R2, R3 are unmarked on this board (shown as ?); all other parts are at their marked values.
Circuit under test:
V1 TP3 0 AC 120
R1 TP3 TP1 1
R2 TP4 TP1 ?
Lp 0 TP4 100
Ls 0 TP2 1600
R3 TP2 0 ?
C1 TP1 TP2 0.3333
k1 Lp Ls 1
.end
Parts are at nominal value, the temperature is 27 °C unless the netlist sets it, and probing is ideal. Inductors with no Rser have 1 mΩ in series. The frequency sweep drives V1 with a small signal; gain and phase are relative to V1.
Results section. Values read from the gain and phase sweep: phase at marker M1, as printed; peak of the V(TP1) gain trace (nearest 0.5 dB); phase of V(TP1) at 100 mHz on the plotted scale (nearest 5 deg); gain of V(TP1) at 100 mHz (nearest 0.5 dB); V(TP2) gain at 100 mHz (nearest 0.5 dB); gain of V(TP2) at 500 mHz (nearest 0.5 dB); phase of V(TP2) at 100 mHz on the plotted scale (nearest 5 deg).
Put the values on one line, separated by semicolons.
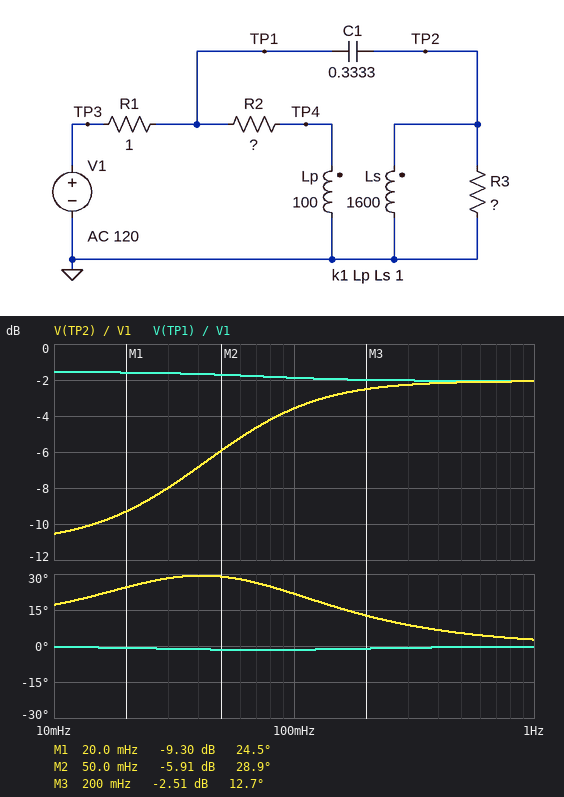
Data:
24.5 deg; -1.5 dB; 0 deg; -2.0 dB; -3.5 dB; -2.0 dB; 20 deg
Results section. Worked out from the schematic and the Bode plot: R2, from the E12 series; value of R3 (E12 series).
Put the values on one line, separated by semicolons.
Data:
4.7 Ω; 6.8 Ω
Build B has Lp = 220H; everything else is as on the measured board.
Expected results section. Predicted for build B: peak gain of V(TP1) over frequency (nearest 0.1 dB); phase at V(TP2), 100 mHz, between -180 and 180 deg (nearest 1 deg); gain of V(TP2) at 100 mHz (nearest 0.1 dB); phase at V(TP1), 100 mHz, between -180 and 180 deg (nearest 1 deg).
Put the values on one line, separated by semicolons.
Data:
-1.4 dB; 18 deg; -3.4 dB; -1 deg
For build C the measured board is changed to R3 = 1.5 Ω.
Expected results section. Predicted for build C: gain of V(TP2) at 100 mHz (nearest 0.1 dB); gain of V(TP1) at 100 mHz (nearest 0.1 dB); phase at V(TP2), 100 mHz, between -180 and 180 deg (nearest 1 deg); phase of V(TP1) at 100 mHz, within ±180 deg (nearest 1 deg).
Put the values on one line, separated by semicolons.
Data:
-12.4 dB; -2.1 dB; 51 deg; -7 deg
